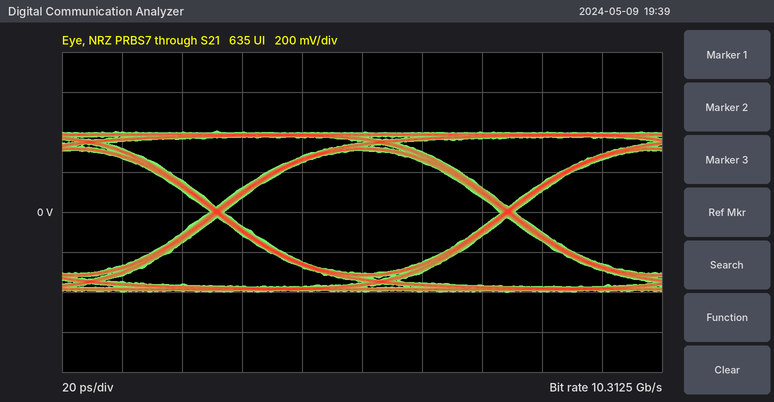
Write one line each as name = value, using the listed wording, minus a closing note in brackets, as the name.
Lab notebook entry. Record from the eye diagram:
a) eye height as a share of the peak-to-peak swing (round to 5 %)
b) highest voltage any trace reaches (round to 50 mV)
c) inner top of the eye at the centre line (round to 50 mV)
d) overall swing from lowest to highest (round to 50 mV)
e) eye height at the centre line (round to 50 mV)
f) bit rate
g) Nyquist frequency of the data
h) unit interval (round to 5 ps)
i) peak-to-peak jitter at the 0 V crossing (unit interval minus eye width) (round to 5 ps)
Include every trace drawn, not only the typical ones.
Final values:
eye height as a share of the peak-to-peak swing = 75 %
highest voltage any trace reaches = 400 mV
inner top of the eye at the centre line = 300 mV
overall swing from lowest to highest = 800 mV
eye height at the centre line = 600 mV
bit rate = 10.3125 Gb/s
Nyquist frequency of the data = 5.15625 GHz
unit interval = 95 ps
peak-to-peak jitter at the 0 V crossing (unit interval minus eye width) = 5 ps
